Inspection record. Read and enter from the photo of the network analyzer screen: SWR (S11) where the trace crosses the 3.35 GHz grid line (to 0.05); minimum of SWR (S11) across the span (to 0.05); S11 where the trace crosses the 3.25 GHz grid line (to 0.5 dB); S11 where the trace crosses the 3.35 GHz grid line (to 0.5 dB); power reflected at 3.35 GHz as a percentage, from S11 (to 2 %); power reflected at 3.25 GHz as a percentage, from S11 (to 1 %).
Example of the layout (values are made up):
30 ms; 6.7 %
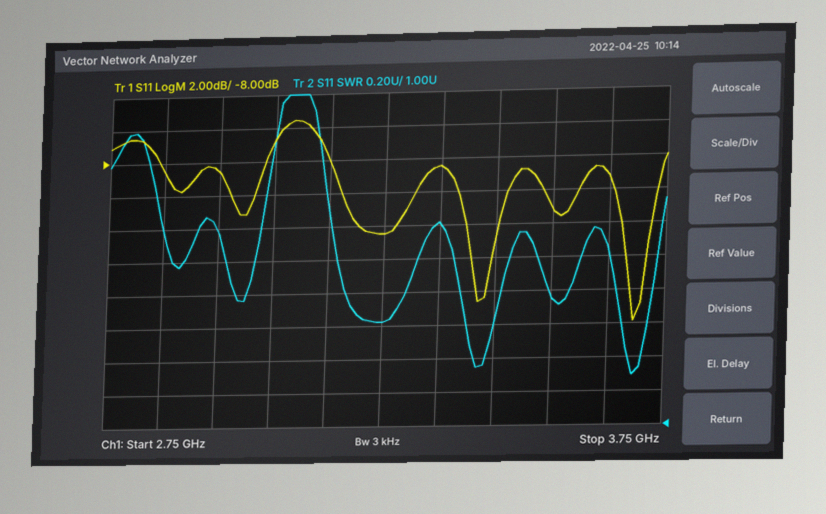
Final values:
2.20; 1.30; -12.5 dB; -8.5 dB; 14 %; 6 %
